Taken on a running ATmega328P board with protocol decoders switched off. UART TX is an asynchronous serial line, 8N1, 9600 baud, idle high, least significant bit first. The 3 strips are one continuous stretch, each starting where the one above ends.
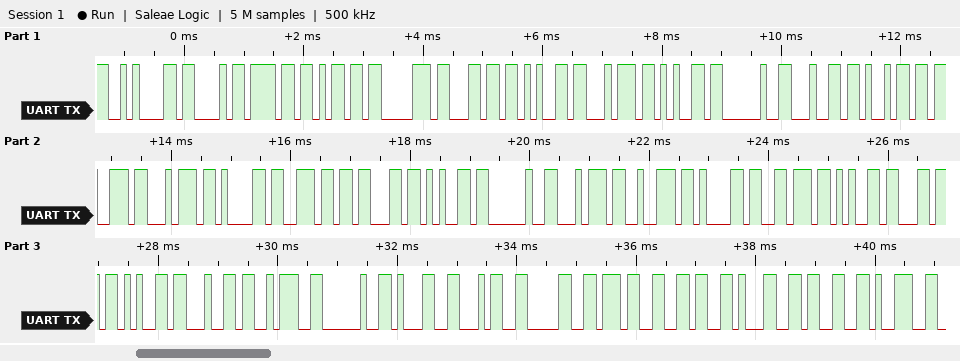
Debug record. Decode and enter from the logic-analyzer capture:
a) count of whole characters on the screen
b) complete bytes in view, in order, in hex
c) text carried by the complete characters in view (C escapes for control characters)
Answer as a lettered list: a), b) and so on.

a) 37
b) 0A 43 6F 6D 70 6C 65 74 65 20 64 69 73 74 61 6E 63 65 20 74 72 61 76 65 6C 65 64 3A 20 31 34 30 37 36 31 33 39
c) "\nComplete distance traveled: 14076139"
